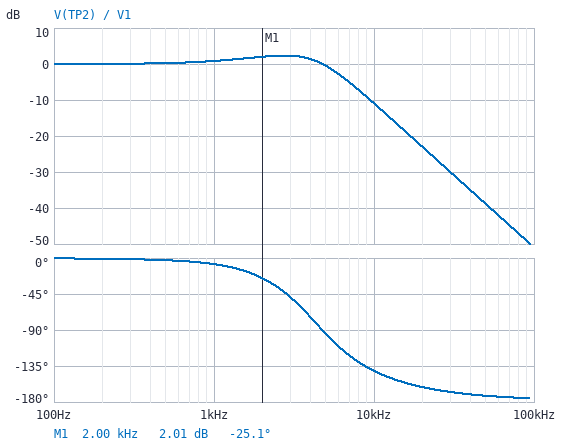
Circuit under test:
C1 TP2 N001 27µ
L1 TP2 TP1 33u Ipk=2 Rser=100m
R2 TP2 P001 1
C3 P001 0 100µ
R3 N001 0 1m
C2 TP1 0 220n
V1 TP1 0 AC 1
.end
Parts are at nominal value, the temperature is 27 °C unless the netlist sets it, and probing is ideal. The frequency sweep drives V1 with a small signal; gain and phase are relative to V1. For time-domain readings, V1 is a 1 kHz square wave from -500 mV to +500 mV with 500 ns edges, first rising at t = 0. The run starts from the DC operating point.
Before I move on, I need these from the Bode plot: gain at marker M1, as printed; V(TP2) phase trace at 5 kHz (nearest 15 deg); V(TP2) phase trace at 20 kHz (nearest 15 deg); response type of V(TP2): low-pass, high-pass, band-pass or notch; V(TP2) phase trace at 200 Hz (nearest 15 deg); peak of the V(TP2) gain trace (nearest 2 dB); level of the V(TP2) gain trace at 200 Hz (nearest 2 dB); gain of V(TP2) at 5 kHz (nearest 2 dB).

2.01 dB
-90 deg
-165 deg
low-pass
0 deg
2 dB
0 dB
0 dB
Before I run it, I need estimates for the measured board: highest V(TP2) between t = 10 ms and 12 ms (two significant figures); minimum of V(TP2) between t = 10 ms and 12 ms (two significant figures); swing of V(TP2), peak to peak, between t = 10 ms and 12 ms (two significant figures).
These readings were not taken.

760 mV
-760 mV
1.5 V
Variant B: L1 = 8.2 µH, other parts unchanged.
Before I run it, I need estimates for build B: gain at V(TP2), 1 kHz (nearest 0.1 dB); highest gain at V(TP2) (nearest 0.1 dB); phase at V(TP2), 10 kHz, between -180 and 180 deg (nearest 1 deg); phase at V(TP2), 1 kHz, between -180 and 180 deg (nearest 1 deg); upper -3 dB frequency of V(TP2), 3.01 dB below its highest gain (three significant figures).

0 dB
3.2 dB
-78 deg
-4 deg
12.8 kHz
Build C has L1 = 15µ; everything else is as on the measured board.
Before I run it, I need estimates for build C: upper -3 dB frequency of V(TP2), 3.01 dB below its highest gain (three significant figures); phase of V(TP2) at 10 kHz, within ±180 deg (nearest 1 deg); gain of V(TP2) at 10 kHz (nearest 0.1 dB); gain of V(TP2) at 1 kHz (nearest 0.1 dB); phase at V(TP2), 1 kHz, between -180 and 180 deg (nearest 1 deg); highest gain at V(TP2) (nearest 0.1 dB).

9.09 kHz
-120 deg
-2.2 dB
0.2 dB
-5 deg
2.4 dB
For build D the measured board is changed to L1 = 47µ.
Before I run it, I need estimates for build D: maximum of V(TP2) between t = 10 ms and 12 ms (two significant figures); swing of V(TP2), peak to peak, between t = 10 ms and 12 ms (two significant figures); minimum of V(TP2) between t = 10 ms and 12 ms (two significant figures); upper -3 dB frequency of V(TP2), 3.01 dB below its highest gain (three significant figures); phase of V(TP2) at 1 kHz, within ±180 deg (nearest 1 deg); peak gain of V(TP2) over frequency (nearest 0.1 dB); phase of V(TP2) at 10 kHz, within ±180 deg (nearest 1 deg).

780 mV
1.6 V
-780 mV
3.71 kHz
-10 deg
2.8 dB
-145 deg
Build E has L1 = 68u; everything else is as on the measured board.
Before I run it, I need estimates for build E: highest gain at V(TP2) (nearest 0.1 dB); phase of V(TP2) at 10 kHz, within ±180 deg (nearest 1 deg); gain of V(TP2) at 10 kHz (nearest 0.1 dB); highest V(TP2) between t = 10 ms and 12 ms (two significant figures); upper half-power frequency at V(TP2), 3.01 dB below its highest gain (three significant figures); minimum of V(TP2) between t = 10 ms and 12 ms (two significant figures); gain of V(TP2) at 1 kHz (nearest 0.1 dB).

3.5 dB
-147 deg
-18.2 dB
820 mV
2.70 kHz
-820 mV
2.1 dB
